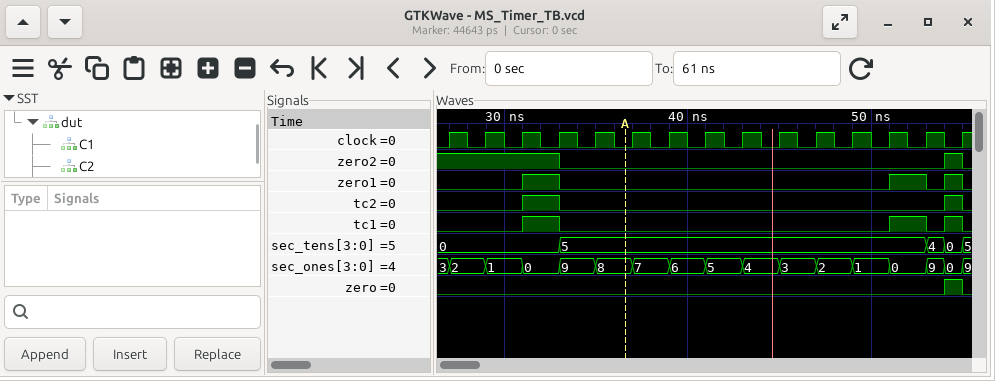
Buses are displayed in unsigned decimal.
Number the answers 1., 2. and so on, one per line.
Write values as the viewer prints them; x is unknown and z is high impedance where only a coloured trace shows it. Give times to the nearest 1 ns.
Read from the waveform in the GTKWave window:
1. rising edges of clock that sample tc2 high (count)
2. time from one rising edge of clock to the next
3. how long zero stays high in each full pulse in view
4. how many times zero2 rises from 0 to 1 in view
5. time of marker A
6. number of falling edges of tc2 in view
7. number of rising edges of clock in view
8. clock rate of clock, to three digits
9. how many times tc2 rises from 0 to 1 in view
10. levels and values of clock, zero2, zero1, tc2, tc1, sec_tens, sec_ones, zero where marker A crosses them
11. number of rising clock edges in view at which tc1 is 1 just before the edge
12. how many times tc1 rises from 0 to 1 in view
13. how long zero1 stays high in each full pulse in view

1. 2
2. 2 ns
3. 1 ns
4. 1
5. 37 ns
6. 2
7. 15
8. 500 MHz
9. 2
10. clock=0, zero2=0, zero1=0, tc2=0, tc1=0, sec_tens=5, sec_ones=8, zero=0
11. 3
12. 3
13. 2 ns, 2 ns, 1 ns
